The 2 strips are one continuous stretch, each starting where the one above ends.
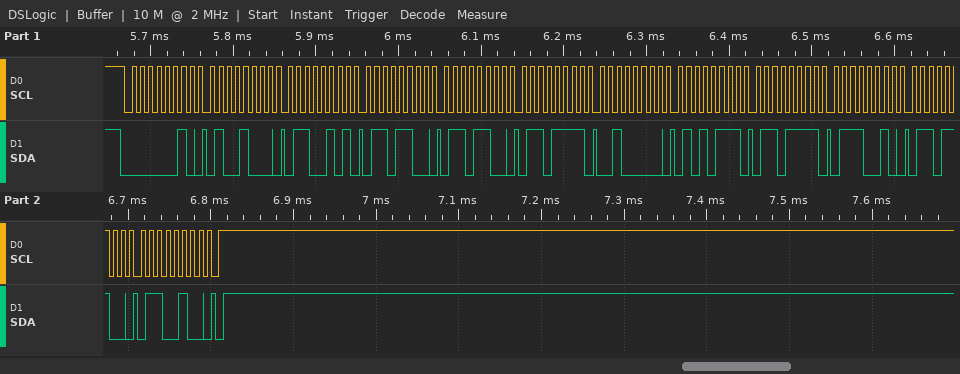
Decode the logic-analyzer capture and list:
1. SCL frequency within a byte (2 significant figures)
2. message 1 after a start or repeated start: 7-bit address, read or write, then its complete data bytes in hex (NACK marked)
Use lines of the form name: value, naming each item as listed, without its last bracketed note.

SCL frequency within a byte: 100 kHz
message 1 after a start or repeated start: 7-bit address, read or write, then its complete data bytes in hex: 0x01 write: 48 65 6C 6C 6F 20 57 6F 72 6C 64
